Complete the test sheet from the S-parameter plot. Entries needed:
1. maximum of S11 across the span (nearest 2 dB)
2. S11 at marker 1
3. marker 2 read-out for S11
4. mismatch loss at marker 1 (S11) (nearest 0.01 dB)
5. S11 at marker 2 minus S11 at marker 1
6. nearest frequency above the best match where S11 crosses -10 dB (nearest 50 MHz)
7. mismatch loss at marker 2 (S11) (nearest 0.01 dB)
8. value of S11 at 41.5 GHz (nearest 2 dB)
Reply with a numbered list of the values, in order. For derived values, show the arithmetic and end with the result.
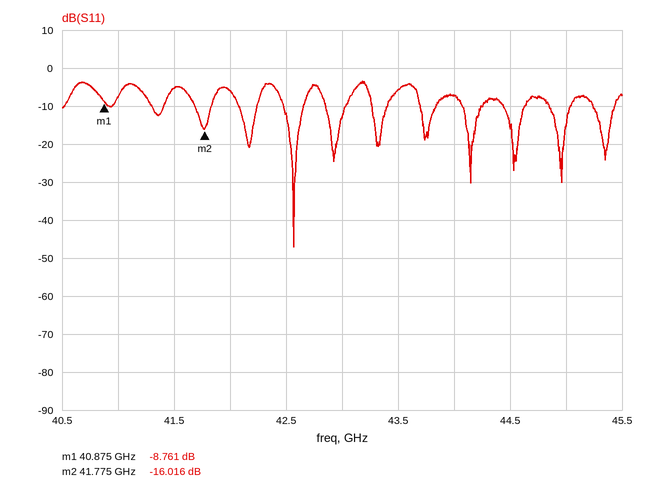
1. -4 dB
2. -8.761 dB
3. -16.016 dB
4. −10 log10(1 − 10^(-8.761/10)) ≈ 0.62 dB
5. -16.016 − (-8.761) = -7.255 dB
6. 42.65 GHz
7. −10 log10(1 − 10^(-16.016/10)) ≈ 0.11 dB
8. -6 dB
